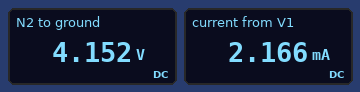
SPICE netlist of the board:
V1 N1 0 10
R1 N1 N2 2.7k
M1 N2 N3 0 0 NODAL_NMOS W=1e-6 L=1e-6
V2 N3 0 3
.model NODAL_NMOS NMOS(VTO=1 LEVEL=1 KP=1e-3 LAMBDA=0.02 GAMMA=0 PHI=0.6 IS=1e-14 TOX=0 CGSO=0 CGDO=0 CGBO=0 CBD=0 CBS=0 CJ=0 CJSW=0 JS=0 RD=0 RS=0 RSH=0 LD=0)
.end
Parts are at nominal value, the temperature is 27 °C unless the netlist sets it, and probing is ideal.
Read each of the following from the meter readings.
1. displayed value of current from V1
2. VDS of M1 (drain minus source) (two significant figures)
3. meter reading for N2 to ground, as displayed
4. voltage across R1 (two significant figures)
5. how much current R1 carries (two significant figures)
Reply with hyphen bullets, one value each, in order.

- 2.166 mA
- 4.2 V
- 4.152 V
- 5.8 V
- 2.2 mA
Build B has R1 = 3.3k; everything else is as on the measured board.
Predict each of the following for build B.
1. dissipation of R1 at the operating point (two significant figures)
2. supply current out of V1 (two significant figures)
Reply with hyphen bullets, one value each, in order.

- 15 mW
- 2.1 mA
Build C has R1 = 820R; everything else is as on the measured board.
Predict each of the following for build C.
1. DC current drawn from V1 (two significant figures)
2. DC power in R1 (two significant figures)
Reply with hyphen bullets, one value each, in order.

- 2.3 mA
- 4.4 mW
